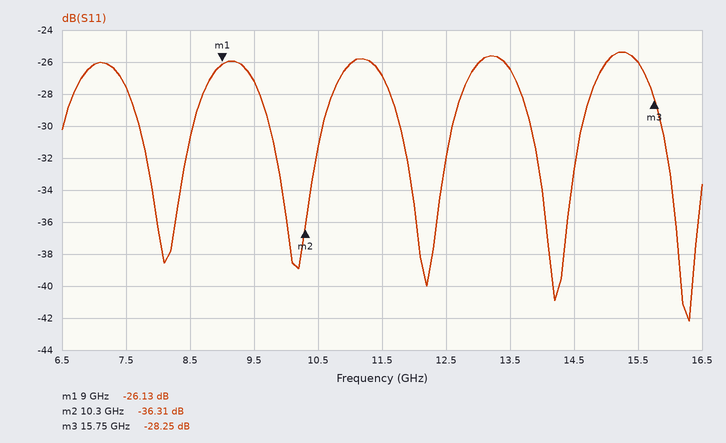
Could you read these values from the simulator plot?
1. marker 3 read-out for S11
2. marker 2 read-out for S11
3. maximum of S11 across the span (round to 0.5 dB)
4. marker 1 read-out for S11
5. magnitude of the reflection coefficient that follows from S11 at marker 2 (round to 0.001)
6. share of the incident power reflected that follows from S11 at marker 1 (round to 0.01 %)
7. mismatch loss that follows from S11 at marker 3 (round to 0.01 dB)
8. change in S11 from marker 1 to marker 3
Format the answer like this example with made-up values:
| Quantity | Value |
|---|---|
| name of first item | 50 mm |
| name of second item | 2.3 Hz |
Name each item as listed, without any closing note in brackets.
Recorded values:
| Quantity | Value |
|---|---|
| marker 3 read-out for S11 | -28.25 dB |
| marker 2 read-out for S11 | -36.31 dB |
| maximum of S11 across the span | -25.5 dB |
| marker 1 read-out for S11 | -26.13 dB |
| magnitude of the reflection coefficient that follows from S11 at marker 2 | 0.015 |
| share of the incident power reflected that follows from S11 at marker 1 | 0.24 % |
| mismatch loss that follows from S11 at marker 3 | 0.01 dB |
| change in S11 from marker 1 to marker 3 | -2.12 dB |
